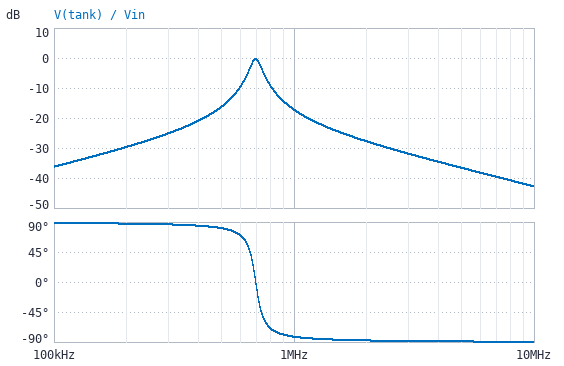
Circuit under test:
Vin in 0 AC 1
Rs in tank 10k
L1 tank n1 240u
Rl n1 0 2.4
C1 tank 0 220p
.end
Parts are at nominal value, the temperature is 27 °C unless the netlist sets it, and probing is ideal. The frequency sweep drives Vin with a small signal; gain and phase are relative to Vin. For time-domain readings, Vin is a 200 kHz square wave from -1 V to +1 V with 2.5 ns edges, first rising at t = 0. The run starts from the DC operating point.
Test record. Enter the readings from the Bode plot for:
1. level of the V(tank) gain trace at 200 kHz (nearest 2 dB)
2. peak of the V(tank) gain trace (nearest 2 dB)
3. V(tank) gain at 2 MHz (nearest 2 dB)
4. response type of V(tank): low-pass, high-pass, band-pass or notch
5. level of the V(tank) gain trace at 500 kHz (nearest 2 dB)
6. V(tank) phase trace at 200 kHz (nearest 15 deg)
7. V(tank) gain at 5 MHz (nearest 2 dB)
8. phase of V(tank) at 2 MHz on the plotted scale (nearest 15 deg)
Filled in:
-30 dB
0 dB
-28 dB
band-pass
-16 dB
90 deg
-36 dB
-90 deg
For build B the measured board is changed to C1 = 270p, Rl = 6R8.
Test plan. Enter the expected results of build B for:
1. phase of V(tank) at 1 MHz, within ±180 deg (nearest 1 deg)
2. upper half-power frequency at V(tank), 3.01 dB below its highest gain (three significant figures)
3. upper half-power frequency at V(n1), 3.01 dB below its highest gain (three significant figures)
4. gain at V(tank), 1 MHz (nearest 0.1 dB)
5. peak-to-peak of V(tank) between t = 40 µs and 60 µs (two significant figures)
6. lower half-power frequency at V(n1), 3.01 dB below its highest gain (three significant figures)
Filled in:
-84 deg
658 kHz
655 kHz
-20.3 dB
730 mV
591 kHz
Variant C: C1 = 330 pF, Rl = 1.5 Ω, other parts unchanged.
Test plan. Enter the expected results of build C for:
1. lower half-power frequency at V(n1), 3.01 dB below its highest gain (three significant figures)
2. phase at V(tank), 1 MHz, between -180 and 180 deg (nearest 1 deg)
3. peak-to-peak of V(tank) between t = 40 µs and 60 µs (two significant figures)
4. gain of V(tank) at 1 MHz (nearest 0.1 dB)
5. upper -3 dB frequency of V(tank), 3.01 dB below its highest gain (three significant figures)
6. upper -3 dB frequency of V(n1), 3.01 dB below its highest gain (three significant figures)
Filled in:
539 kHz
-86 deg
560 mV
-23.0 dB
591 kHz
589 kHz
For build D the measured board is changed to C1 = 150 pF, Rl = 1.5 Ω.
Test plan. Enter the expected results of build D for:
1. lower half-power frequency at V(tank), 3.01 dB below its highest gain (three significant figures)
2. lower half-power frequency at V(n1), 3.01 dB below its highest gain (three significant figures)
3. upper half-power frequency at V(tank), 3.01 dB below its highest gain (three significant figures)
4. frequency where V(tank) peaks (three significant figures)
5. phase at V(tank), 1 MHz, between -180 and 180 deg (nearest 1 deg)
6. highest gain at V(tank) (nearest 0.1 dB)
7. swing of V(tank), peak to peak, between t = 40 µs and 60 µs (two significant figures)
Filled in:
787 kHz
780 kHz
894 kHz
839 kHz
-70 deg
-0.1 dB
330 mV
